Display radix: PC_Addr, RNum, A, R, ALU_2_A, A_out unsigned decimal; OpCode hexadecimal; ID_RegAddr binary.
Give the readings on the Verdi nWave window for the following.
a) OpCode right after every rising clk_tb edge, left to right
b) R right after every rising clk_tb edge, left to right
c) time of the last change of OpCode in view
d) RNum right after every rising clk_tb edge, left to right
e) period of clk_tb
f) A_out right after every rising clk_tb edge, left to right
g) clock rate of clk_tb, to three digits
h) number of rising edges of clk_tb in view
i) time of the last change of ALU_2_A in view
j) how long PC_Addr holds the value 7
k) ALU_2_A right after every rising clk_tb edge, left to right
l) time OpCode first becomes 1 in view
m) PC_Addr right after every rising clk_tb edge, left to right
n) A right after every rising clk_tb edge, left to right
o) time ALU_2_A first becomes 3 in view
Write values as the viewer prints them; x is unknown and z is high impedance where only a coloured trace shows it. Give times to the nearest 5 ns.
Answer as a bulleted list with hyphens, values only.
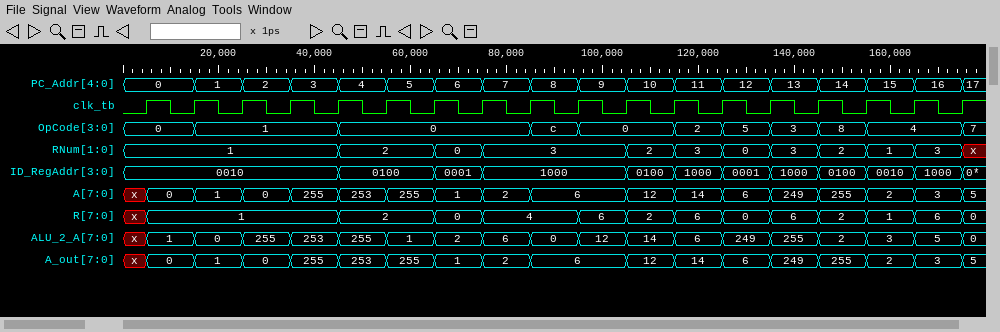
- 0, 1, 1, 1, 0, 0, 0, 0, c, 0, 0, 2, 5, 3, 8, 4, 4, 7
- 1, 1, 1, 1, 2, 2, 0, 4, 4, 6, 2, 6, 0, 6, 2, 1, 6, 0
- 175 ns
- 1, 1, 1, 1, 2, 2, 0, 3, 3, 3, 2, 3, 0, 3, 2, 1, 3, x
- 10 ns
- 0, 1, 0, 255, 253, 255, 1, 2, 6, 6, 12, 14, 6, 249, 255, 2, 3, 5
- 100 MHz
- 18
- 175 ns
- 10 ns
- 1, 0, 255, 253, 255, 1, 2, 6, 0, 12, 14, 6, 249, 255, 2, 3, 5, 0
- 15 ns
- 0, 1, 2, 3, 4, 5, 6, 7, 8, 9, 10, 11, 12, 13, 14, 15, 16, 17
- 0, 1, 0, 255, 253, 255, 1, 2, 6, 6, 12, 14, 6, 249, 255, 2, 3, 5
- 155 ns
